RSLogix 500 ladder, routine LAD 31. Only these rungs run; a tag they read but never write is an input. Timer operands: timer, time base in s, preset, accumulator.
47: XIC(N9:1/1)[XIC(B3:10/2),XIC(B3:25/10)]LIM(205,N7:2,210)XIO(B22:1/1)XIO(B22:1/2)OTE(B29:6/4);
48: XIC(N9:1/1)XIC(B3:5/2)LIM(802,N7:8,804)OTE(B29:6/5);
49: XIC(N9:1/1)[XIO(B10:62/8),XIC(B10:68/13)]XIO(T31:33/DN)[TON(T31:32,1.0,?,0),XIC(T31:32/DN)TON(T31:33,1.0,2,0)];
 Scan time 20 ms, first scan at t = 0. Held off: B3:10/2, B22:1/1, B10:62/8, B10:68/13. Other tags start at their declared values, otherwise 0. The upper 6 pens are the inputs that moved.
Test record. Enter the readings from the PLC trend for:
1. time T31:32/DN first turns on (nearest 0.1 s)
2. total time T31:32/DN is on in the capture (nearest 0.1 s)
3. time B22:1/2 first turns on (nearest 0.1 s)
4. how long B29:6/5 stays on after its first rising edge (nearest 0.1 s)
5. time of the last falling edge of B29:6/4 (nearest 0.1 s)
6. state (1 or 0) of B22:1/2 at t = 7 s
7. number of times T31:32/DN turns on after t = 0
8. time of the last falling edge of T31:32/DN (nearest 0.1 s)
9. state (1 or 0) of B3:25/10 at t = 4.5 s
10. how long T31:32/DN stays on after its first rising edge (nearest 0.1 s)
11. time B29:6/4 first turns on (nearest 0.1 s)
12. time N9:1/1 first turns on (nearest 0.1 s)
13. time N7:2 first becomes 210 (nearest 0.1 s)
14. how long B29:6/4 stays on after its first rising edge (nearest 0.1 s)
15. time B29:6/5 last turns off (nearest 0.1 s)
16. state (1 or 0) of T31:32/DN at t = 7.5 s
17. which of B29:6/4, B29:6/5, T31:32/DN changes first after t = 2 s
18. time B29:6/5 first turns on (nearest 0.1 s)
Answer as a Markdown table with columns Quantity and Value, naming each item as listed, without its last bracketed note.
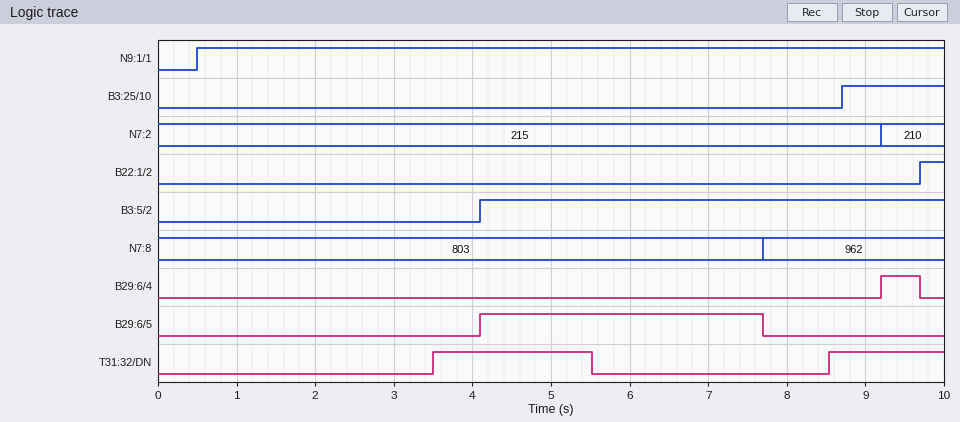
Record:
| Quantity | Value |
|---|---|
| time T31:32/DN first turns on | 3.5 s |
| total time T31:32/DN is on in the capture | 3.5 s |
| time B22:1/2 first turns on | 9.7 s |
| how long B29:6/5 stays on after its first rising edge | 3.6 s |
| time of the last falling edge of B29:6/4 | 9.7 s |
| state (1 or 0) of B22:1/2 at t = 7 s | 0 |
| number of times T31:32/DN turns on after t = 0 | 2 |
| time of the last falling edge of T31:32/DN | 5.5 s |
| state (1 or 0) of B3:25/10 at t = 4.5 s | 0 |
| how long T31:32/DN stays on after its first rising edge | 2.0 s |
| time B29:6/4 first turns on | 9.2 s |
| time N9:1/1 first turns on | 0.5 s |
| time N7:2 first becomes 210 | 9.2 s |
| how long B29:6/4 stays on after its first rising edge | 0.5 s |
| time B29:6/5 last turns off | 7.7 s |
| state (1 or 0) of T31:32/DN at t = 7.5 s | 0 |
| which of B29:6/4, B29:6/5, T31:32/DN changes first after t = 2 s | T31:32/DN |
| time B29:6/5 first turns on | 4.1 s |
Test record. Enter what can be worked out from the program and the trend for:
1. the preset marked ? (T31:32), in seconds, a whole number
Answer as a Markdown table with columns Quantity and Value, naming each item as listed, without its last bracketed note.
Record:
| Quantity | Value |
|---|---|
| the preset marked ? (T31:32), in seconds, a whole number | 3 s |
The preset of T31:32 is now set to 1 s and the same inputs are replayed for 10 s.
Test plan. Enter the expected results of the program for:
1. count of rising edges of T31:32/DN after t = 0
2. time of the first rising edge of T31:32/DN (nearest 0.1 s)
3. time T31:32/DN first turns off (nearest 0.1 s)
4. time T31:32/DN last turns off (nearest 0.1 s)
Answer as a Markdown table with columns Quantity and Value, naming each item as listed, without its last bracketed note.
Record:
| Quantity | Value |
|---|---|
| count of rising edges of T31:32/DN after t = 0 | 3 |
| time of the first rising edge of T31:32/DN | 1.5 s |
| time T31:32/DN first turns off | 3.5 s |
| time T31:32/DN last turns off | 9.6 s |
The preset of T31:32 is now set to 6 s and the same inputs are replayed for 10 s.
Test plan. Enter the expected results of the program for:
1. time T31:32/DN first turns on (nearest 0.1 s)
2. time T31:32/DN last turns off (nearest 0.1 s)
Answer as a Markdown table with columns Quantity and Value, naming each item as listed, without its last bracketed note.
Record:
| Quantity | Value |
|---|---|
| time T31:32/DN first turns on | 6.5 s |
| time T31:32/DN last turns off | 8.5 s |
